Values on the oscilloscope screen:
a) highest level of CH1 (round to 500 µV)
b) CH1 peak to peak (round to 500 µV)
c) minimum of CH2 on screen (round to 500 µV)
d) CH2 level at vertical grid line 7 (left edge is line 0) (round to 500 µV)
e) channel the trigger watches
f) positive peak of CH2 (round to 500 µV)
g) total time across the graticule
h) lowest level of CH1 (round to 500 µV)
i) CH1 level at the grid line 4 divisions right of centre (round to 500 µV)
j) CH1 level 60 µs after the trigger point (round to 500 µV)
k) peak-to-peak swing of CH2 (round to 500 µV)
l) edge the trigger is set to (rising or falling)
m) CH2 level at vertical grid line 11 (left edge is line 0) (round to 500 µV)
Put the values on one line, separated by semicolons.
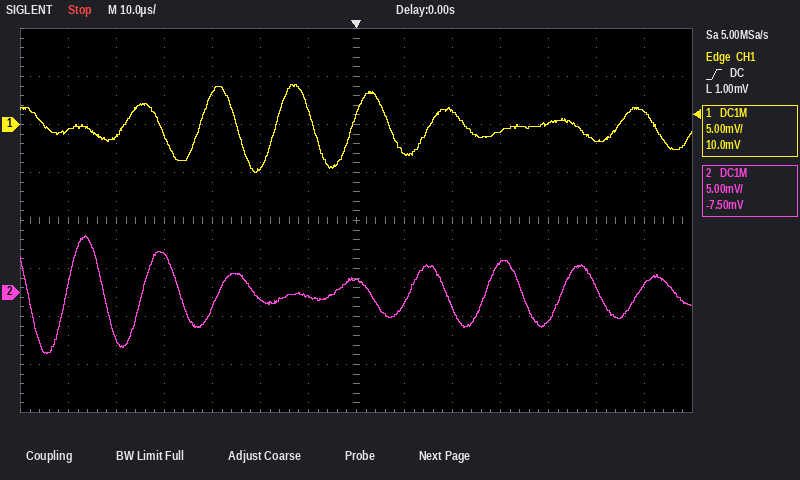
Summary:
4.0 mV; 9.0 mV; -6.5 mV; 1.5 mV; CH1; 6.0 mV; 140 µs; -5.0 mV; 0.0 mV; 1.5 mV; 12.5 mV; rising; -3.0 mV
